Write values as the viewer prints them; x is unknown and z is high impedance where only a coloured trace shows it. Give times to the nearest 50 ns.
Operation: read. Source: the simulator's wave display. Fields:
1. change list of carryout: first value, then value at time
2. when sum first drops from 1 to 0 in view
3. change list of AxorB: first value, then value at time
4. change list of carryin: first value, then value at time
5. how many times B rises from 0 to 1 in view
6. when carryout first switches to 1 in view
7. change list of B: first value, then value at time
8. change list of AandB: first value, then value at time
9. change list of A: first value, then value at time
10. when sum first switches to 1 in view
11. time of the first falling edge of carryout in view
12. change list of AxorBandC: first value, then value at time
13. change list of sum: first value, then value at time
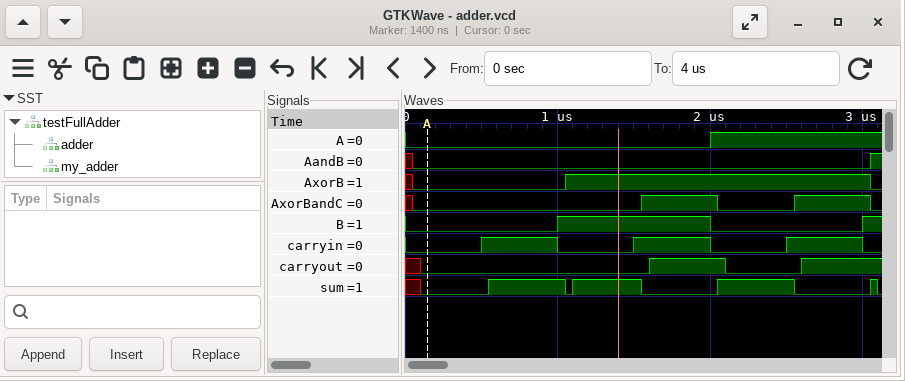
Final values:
x, 0 at 100 ns, 1 at 1600 ns, 0 at 2100 ns, 1 at 2600 ns
1050 ns
x, 0 at 50 ns, 1 at 1050 ns, 0 at 3050 ns
0, 1 at 500 ns, 0 at 1000 ns, 1 at 1500 ns, 0 at 2000 ns, 1 at 2500 ns, 0 at 3000 ns
2
1600 ns
0, 1 at 1000 ns, 0 at 2000 ns, 1 at 3000 ns
x, 0 at 50 ns, 1 at 3050 ns
0, 1 at 2000 ns
550 ns
2100 ns
x, 0 at 50 ns, 1 at 1550 ns, 0 at 2050 ns, 1 at 2550 ns, 0 at 3050 ns
x, 0 at 100 ns, 1 at 550 ns, 0 at 1050 ns, 1 at 1100 ns, 0 at 1550 ns, 1 at 2050 ns, 0 at 2550 ns, 1 at 3050 ns, 0 at 3100 ns
